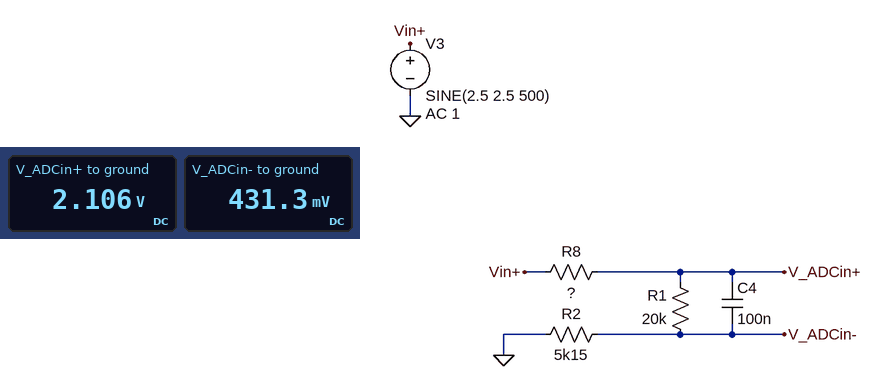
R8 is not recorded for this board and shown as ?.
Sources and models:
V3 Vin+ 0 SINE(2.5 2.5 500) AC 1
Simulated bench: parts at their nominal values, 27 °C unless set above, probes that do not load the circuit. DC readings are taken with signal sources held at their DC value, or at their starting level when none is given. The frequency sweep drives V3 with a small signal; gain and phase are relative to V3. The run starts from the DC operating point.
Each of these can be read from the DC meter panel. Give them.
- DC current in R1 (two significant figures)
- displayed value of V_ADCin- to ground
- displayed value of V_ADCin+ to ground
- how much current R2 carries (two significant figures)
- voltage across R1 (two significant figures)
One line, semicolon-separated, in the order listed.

84 µA; 431.3 mV; 2.106 V; 84 µA; 1.7 V
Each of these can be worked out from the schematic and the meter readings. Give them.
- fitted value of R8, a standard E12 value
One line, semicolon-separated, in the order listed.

4.7 kΩ
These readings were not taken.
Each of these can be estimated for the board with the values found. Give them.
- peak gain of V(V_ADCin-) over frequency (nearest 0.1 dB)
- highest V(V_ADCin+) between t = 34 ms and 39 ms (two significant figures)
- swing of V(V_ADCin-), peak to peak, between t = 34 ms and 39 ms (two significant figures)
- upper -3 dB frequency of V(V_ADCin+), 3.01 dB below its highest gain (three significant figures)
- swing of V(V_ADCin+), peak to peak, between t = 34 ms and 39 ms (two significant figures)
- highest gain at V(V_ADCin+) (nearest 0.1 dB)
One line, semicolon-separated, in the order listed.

-5.6 dB; 3.6 V; 2.4 V; 503 Hz; 3.0 V; -1.5 dB
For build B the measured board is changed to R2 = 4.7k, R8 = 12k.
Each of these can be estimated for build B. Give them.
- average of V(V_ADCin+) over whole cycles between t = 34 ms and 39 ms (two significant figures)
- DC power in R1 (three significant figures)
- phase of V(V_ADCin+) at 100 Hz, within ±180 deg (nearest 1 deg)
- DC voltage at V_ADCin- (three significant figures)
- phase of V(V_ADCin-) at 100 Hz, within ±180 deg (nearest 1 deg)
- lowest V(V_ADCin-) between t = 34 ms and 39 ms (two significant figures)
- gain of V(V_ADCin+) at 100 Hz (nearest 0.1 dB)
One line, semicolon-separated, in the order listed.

1.7 V; 92.8 µW; -16 deg; 320 mV; 22 deg; -350 mV; -4.4 dB
